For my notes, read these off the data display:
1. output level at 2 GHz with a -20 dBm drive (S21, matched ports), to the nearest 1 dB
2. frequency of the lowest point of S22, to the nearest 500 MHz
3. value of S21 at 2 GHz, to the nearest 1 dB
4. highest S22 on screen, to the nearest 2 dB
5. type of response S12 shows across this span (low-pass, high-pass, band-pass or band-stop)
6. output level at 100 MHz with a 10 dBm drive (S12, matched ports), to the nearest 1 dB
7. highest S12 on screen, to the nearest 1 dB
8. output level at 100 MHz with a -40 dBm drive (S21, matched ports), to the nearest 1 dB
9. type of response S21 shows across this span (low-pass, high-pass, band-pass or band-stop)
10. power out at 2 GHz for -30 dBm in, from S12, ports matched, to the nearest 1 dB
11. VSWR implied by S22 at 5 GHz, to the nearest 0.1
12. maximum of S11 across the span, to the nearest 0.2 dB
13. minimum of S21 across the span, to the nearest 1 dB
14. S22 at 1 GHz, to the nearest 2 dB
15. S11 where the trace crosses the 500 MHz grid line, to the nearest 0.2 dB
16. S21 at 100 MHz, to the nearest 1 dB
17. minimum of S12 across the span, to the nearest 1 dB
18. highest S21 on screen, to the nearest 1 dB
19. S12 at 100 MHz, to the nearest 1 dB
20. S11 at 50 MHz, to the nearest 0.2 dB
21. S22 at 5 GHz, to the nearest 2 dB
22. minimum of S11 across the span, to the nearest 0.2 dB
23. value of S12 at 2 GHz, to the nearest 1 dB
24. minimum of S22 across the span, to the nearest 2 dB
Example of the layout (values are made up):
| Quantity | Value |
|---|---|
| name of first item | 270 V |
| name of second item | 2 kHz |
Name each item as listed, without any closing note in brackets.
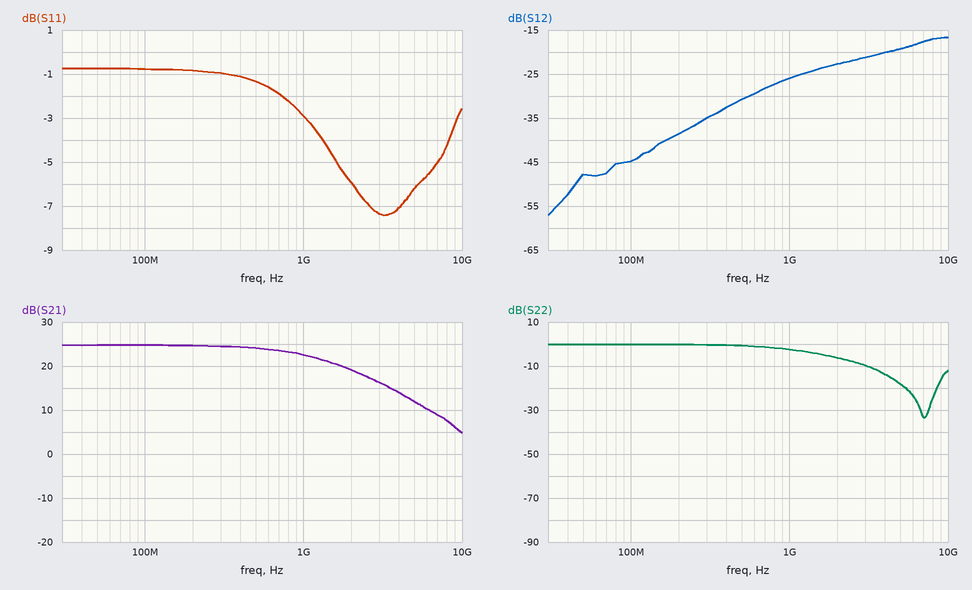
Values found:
| Quantity | Value |
|---|---|
| output level at 2 GHz with a -20 dBm drive (S21, matched ports), to the nearest 1 dB | -1 dBm |
| frequency of the lowest point of S22, to the nearest 500 MHz | 7.0 GHz |
| value of S21 at 2 GHz, to the nearest 1 dB | 19 dB |
| highest S22 on screen, to the nearest 2 dB | 0 dB |
| type of response S12 shows across this span | high-pass |
| output level at 100 MHz with a 10 dBm drive (S12, matched ports), to the nearest 1 dB | -35 dBm |
| highest S12 on screen, to the nearest 1 dB | -17 dB |
| output level at 100 MHz with a -40 dBm drive (S21, matched ports), to the nearest 1 dB | -15 dBm |
| type of response S21 shows across this span | low-pass |
| power out at 2 GHz for -30 dBm in, from S12, ports matched, to the nearest 1 dB | -53 dBm |
| VSWR implied by S22 at 5 GHz, to the nearest 0.1 | 1.3 |
| maximum of S11 across the span, to the nearest 0.2 dB | -0.8 dB |
| minimum of S21 across the span, to the nearest 1 dB | 5 dB |
| S22 at 1 GHz, to the nearest 2 dB | -2 dB |
| S11 where the trace crosses the 500 MHz grid line, to the nearest 0.2 dB | -1.4 dB |
| S21 at 100 MHz, to the nearest 1 dB | 25 dB |
| minimum of S12 across the span, to the nearest 1 dB | -57 dB |
| highest S21 on screen, to the nearest 1 dB | 25 dB |
| S12 at 100 MHz, to the nearest 1 dB | -45 dB |
| S11 at 50 MHz, to the nearest 0.2 dB | -0.8 dB |
| S22 at 5 GHz, to the nearest 2 dB | -18 dB |
| minimum of S11 across the span, to the nearest 0.2 dB | -7.4 dB |
| value of S12 at 2 GHz, to the nearest 1 dB | -23 dB |
| minimum of S22 across the span, to the nearest 2 dB | -34 dB |
